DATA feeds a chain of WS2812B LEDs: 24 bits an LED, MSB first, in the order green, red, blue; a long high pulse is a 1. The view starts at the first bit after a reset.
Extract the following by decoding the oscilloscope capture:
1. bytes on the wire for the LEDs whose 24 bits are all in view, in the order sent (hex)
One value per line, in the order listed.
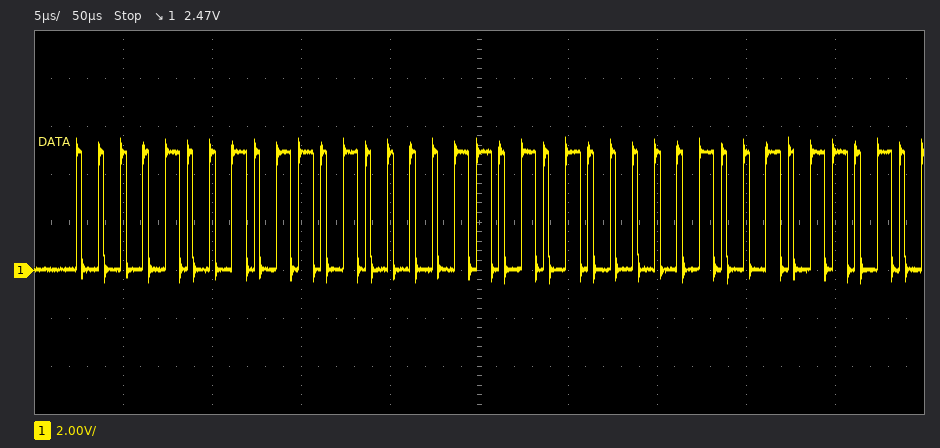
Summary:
09 68 6A
